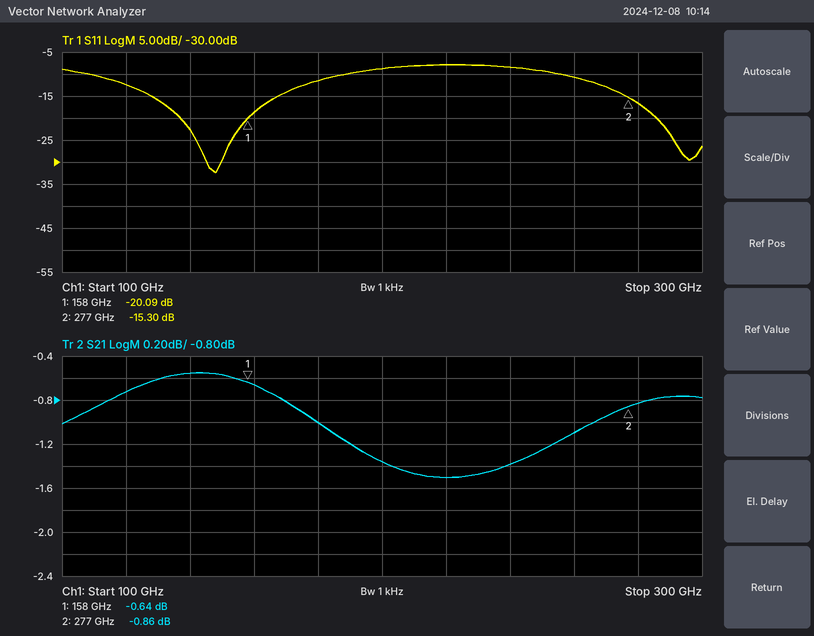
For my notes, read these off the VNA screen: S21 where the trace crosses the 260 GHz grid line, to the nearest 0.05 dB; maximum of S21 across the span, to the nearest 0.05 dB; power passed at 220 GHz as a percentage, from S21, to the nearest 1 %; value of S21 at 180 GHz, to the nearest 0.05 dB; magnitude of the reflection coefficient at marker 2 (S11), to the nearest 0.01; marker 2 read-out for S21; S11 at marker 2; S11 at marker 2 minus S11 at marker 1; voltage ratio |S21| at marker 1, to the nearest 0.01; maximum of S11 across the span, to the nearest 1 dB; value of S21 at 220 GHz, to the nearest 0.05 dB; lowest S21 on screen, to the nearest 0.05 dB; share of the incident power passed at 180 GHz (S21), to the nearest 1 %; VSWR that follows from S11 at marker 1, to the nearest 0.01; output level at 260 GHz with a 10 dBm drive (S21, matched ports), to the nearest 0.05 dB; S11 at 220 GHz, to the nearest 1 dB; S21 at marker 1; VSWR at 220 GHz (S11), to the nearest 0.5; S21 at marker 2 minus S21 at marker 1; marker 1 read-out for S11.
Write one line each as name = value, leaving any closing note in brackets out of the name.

S21 where the trace crosses the 260 GHz grid line, to the nearest 0.05 dB = -1.10 dB
maximum of S21 across the span, to the nearest 0.05 dB = -0.55 dB
power passed at 220 GHz as a percentage, from S21, to the nearest 1 % = 71 %
value of S21 at 180 GHz, to the nearest 0.05 dB = -1.00 dB
magnitude of the reflection coefficient at marker 2 (S11), to the nearest 0.01 = 0.17
marker 2 read-out for S21 = -0.86 dB
S11 at marker 2 = -15.30 dB
S11 at marker 2 minus S11 at marker 1 = 4.79 dB
voltage ratio |S21| at marker 1, to the nearest 0.01 = 0.93
maximum of S11 across the span, to the nearest 1 dB = -8 dB
value of S21 at 220 GHz, to the nearest 0.05 dB = -1.50 dB
lowest S21 on screen, to the nearest 0.05 dB = -1.50 dB
share of the incident power passed at 180 GHz (S21), to the nearest 1 % = 79 %
VSWR that follows from S11 at marker 1, to the nearest 0.01 = 1.22
output level at 260 GHz with a 10 dBm drive (S21, matched ports), to the nearest 0.05 dB = 8.90 dBm
S11 at 220 GHz, to the nearest 1 dB = -8 dB
S21 at marker 1 = -0.64 dB
VSWR at 220 GHz (S11), to the nearest 0.5 = 2.5
S21 at marker 2 minus S21 at marker 1 = -0.22 dB
marker 1 read-out for S11 = -20.09 dB
